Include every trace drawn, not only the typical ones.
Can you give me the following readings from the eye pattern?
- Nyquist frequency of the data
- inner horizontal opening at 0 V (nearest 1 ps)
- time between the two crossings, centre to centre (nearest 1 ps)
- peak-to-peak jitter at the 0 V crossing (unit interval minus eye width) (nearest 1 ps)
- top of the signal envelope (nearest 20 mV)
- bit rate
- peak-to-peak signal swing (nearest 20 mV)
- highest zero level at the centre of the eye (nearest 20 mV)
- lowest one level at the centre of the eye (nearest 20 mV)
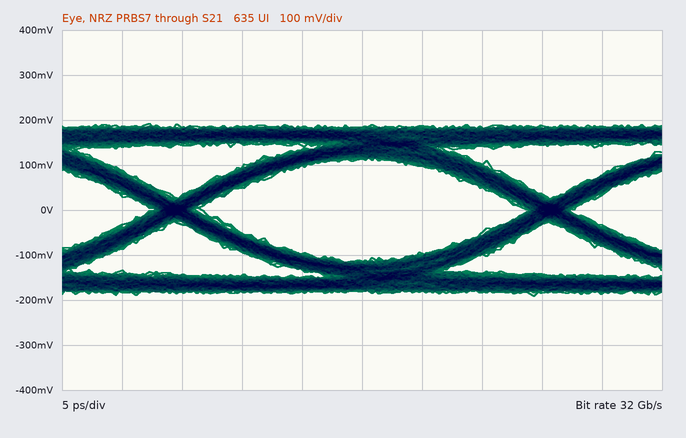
16 GHz
27 ps
31 ps
4 ps
200 mV
32 Gb/s
380 mV
-120 mV
120 mV
